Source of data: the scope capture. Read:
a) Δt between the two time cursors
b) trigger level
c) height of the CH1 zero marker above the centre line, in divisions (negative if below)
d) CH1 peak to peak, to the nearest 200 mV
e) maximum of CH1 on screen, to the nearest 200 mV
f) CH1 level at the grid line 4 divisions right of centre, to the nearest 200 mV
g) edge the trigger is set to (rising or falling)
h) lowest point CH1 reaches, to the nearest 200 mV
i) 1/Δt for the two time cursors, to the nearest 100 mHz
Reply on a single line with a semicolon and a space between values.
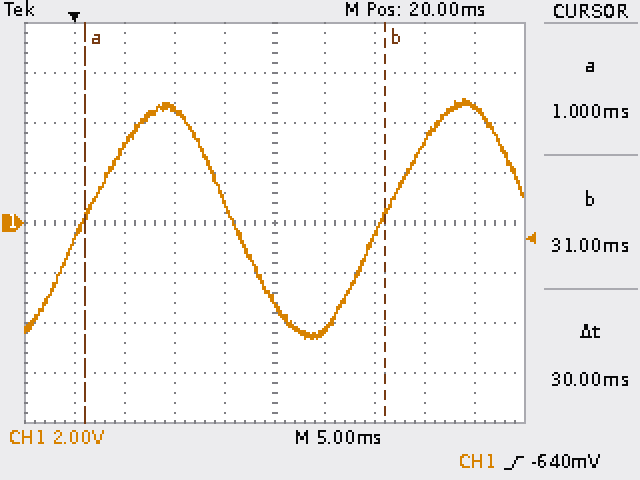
30 ms; -640 mV; 0.0 div; 9.6 V; 5.0 V; 4.6 V; rising; -4.6 V; 33.3 Hz
